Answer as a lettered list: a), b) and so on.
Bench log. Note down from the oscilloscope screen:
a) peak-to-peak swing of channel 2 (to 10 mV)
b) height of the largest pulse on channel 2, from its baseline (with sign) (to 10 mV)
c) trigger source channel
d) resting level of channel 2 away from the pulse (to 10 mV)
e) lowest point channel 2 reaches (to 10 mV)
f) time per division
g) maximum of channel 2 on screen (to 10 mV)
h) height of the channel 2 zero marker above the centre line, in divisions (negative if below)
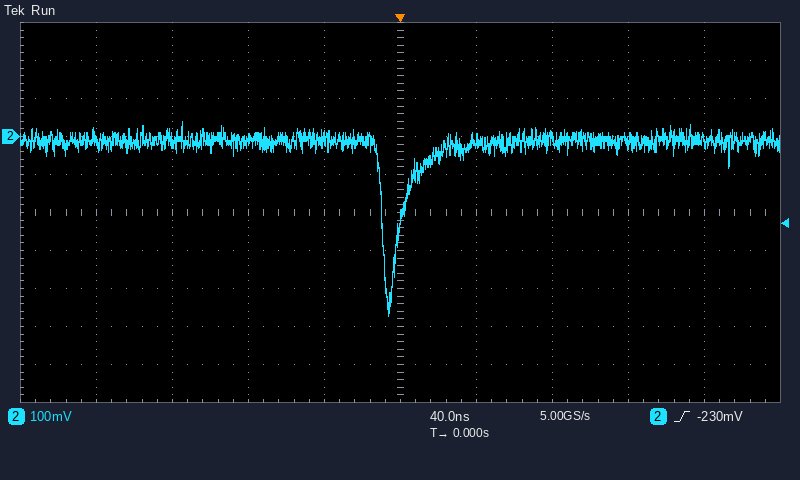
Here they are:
a) 510 mV
b) -460 mV
c) channel 2
d) -10 mV
e) -470 mV
f) 40 ns
g) 40 mV
h) +2.0 div
